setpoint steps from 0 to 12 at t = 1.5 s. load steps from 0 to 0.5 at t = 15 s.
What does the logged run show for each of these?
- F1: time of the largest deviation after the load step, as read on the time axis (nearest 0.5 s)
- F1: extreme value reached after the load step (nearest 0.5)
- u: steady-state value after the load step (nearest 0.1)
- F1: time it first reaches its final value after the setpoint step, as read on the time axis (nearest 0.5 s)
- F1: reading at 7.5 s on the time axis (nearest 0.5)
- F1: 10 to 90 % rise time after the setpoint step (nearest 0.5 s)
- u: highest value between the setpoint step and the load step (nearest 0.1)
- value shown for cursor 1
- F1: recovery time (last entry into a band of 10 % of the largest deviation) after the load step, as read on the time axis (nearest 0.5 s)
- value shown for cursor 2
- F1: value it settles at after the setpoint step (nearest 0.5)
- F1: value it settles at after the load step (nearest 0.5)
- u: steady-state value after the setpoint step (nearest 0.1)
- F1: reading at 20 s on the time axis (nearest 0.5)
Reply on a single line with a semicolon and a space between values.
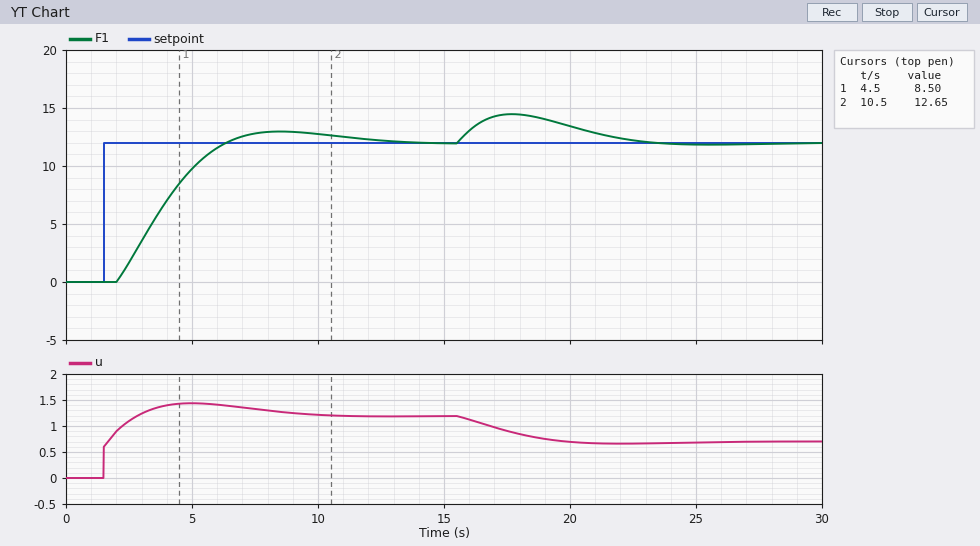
17.5 s; 14.5; 0.7; 6.5 s; 13.0; 3.0 s; 1.4; 8.50; 22.5 s; 12.65; 12.0; 12.0; 1.2; 13.5
